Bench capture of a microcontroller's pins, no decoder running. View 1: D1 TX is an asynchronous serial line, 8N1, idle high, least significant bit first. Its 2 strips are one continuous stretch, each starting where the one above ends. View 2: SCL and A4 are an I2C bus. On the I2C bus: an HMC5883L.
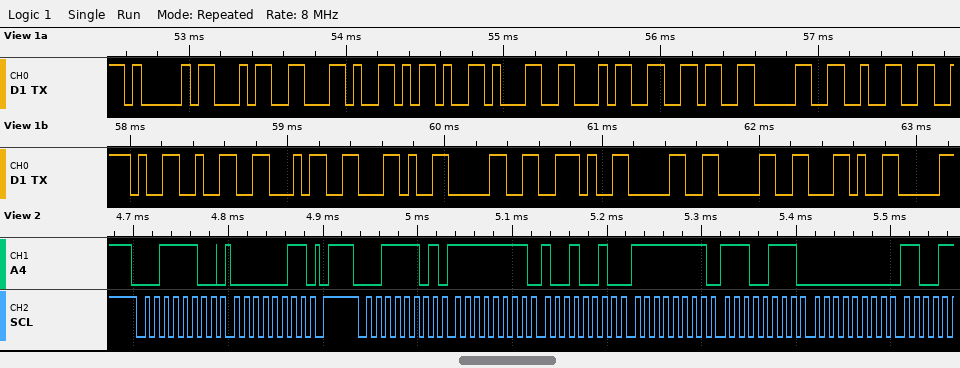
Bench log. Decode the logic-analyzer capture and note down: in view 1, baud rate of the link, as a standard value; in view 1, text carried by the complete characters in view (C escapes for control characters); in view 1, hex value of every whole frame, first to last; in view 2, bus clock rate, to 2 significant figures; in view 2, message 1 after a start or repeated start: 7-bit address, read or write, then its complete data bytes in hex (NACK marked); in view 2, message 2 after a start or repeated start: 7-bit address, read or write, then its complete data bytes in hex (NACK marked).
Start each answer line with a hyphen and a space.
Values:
- 19200 baud
- "A4,-14602.24,0.00,"
- 0x41 0x34 0x2C 0x2D 0x31 0x34 0x36 0x30 0x32 0x2E 0x32 0x34 0x2C 0x30 0x2E 0x30 0x30 0x2C
- 100 kHz
- 0x1E write: 03
- 0x1E read: FF 92 FF E7 00
